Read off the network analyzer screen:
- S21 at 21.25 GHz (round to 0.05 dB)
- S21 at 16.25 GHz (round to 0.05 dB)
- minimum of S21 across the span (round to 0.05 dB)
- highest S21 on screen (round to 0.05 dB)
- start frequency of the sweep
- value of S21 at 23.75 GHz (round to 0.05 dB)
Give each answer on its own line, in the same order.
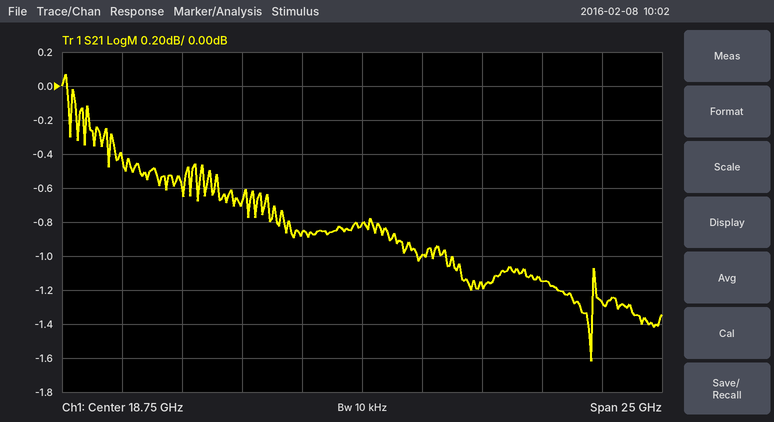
-1.00 dB
-0.85 dB
-1.60 dB
0.05 dB
6.25 GHz
-1.15 dB
